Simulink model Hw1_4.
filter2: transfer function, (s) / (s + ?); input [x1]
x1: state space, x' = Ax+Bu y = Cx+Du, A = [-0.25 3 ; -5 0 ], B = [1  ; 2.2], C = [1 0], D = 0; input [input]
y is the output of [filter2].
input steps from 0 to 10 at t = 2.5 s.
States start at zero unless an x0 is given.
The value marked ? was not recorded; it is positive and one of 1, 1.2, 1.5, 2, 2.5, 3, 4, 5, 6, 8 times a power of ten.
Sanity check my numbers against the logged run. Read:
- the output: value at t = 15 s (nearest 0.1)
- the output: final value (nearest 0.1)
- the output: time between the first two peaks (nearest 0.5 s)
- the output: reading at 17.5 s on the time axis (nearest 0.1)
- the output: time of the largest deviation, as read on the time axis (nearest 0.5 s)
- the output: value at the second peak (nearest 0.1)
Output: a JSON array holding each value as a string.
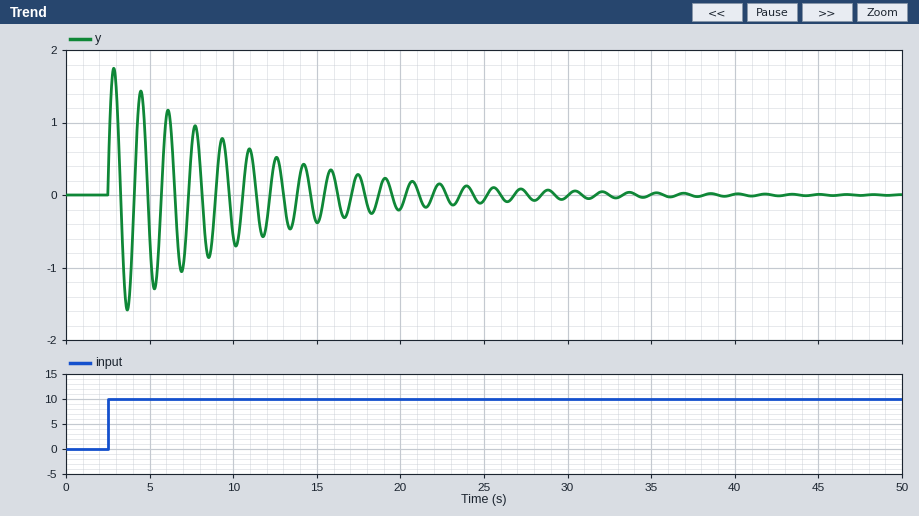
["-0.4", "0.0", "1.5 s", "0.3", "3.0 s", "1.4"]
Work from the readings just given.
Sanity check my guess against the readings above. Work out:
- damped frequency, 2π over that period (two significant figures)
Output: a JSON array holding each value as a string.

["4.2 rad/s"]
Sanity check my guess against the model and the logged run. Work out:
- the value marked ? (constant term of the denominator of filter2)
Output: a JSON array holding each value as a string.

["10"]
